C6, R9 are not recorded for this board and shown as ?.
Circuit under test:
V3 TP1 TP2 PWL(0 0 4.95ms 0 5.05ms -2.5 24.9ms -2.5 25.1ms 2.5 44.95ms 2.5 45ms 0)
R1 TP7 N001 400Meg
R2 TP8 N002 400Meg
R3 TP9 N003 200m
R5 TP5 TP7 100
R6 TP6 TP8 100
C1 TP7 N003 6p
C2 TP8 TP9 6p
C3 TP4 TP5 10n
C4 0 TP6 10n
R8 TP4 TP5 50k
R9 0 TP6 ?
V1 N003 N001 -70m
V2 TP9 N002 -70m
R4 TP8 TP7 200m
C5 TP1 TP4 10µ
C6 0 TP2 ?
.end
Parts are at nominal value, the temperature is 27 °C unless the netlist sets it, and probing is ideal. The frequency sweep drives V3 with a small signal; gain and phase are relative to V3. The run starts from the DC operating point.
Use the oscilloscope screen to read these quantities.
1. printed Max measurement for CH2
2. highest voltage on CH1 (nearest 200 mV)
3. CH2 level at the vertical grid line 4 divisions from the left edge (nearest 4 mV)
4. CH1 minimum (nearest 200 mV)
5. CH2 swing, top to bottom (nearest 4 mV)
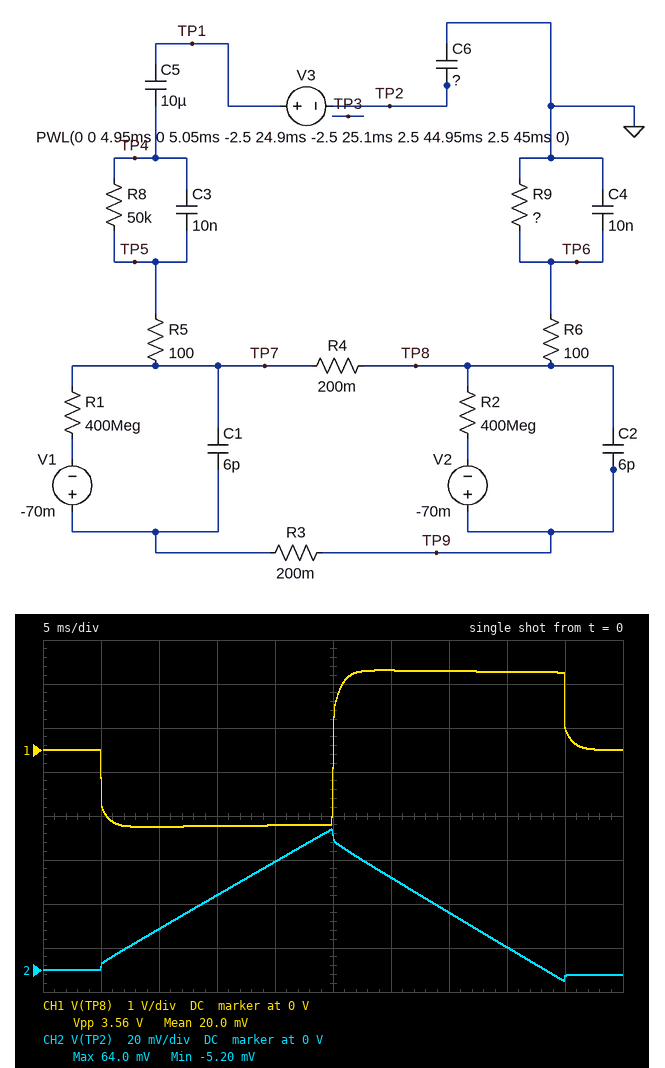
64.0 mV
1.8 V
48 mV
-1.8 V
68 mV
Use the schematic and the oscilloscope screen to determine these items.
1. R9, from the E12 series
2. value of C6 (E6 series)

120 kΩ
4.7 µF
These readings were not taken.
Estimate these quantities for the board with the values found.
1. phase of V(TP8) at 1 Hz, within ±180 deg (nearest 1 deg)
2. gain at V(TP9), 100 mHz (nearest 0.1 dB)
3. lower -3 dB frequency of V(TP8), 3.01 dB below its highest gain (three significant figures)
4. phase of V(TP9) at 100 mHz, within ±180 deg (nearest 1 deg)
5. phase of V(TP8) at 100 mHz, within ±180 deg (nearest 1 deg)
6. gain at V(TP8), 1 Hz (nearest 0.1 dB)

16 deg
-12.8 dB
291 mHz
71 deg
71 deg
-3.4 dB
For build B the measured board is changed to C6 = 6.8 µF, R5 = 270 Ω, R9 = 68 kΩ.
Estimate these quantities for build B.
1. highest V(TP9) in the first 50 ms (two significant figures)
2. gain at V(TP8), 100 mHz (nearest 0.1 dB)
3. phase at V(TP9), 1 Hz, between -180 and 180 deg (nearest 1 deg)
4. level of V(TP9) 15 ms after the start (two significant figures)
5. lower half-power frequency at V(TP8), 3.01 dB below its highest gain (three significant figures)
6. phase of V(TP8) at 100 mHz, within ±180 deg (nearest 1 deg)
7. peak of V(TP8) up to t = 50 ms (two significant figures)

1.4 V
-15.6 dB
18 deg
-1.5 V
331 mHz
73 deg
1.5 V
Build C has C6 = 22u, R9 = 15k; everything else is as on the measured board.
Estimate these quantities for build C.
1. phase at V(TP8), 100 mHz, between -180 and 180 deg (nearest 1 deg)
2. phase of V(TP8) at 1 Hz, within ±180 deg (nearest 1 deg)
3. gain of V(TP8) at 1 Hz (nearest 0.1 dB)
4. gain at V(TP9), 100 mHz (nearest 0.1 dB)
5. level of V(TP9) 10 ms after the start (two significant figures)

74 deg
20 deg
-13.2 dB
-24.0 dB
-640 mV
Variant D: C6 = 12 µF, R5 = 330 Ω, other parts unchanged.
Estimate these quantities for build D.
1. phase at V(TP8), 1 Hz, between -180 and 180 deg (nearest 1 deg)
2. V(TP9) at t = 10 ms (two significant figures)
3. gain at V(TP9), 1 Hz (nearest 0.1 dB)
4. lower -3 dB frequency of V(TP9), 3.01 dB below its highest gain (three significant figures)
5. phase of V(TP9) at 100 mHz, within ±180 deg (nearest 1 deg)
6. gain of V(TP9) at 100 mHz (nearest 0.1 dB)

10 deg
-1.8 V
-3.2 dB
171 mHz
60 deg
-9.0 dB
